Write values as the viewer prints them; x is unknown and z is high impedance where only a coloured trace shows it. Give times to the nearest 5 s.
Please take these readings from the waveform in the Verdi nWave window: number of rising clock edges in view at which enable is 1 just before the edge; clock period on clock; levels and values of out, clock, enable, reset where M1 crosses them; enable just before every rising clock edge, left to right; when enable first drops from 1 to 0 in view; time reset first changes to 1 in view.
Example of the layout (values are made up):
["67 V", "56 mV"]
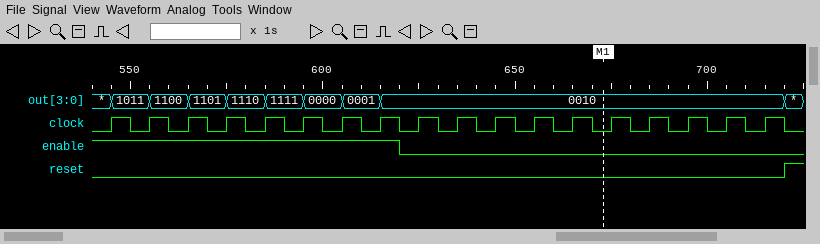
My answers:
["8", "10 s", "out=0010, clock=0, enable=0, reset=0", "1 1 1 1 1 1 1 1 0 0 0 0 0 0 0 0 0 0", "620 s", "720 s"]
